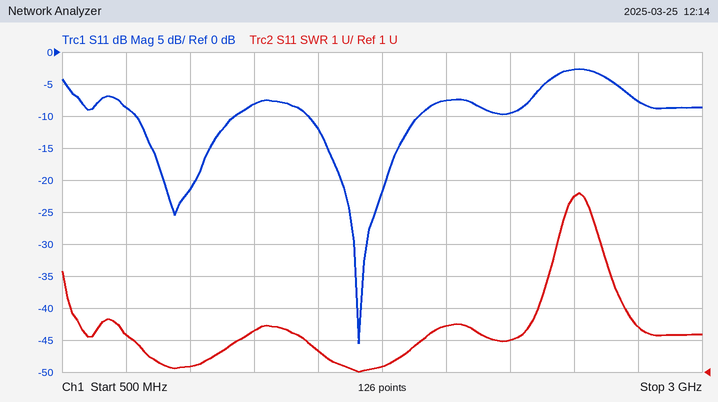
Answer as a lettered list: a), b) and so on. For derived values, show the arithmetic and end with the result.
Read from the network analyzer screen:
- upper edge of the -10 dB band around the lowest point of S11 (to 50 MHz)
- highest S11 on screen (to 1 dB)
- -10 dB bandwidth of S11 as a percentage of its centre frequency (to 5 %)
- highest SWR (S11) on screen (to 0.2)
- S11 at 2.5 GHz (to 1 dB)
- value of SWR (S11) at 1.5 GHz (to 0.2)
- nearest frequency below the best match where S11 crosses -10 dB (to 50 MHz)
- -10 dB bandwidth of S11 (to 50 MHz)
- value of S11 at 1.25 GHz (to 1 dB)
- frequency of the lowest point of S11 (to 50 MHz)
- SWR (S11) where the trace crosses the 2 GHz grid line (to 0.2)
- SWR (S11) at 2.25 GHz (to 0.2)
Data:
a) 1.90 GHz
b) -3 dB
c) 450 MHz / 1.675 GHz ≈ 26.9 %, so 25 % to the nearest 5 %
d) 6.6
e) -3 dB
f) 1.6
g) 1.45 GHz
h) 1.90 GHz − 1.45 GHz = 450 MHz
i) -8 dB
j) 1.65 GHz
k) 2.4
l) 2.0
